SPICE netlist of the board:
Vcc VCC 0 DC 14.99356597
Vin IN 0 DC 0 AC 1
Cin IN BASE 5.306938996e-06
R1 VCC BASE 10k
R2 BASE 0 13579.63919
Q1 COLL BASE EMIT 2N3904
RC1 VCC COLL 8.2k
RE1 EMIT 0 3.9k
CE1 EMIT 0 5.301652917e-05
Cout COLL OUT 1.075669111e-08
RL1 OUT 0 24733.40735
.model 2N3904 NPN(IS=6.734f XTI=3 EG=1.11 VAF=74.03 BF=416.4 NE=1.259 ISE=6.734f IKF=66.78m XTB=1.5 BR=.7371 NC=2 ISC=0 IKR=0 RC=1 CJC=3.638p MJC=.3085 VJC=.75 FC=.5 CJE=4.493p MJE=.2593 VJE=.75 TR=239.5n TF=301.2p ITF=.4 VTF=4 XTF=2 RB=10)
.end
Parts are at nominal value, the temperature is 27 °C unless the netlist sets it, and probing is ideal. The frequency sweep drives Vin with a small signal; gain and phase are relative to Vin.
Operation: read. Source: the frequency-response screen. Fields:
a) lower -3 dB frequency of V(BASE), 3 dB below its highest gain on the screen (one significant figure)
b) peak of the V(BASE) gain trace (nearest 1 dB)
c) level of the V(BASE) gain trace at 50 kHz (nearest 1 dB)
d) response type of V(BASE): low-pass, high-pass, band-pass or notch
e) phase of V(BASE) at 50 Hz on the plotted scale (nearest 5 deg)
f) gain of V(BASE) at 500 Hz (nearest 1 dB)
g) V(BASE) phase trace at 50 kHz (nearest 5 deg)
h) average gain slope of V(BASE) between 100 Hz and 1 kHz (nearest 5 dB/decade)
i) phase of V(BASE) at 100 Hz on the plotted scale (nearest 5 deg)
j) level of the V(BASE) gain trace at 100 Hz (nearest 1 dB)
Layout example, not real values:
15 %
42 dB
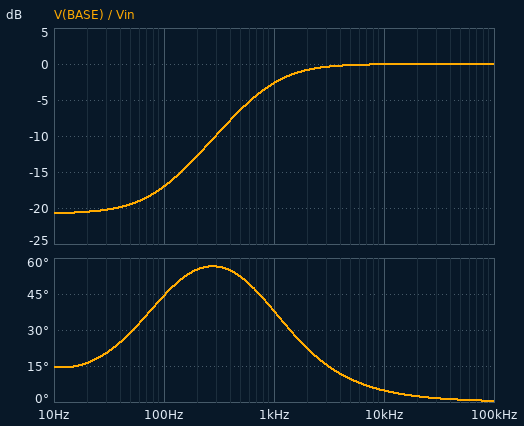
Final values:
900 Hz
0 dB
0 dB
high-pass
30 deg
-6 dB
0 deg
15 dB/decade
45 deg
-17 dB
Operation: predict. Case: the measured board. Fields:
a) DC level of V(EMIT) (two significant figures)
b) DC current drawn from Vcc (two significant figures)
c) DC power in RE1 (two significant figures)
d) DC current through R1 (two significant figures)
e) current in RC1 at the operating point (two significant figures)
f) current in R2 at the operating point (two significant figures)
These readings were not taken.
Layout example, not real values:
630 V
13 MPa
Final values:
5.8 V
2.0 mA
8.6 mW
850 µA
1.1 mA
480 µA
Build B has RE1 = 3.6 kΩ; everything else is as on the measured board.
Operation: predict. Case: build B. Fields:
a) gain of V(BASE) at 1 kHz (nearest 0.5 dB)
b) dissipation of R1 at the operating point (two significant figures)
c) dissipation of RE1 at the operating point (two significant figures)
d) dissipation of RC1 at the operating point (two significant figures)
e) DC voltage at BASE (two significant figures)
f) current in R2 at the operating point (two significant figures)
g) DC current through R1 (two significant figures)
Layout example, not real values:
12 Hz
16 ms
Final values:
-3.0 dB
7.6 mW
8.7 mW
11 mW
6.3 V
460 µA
870 µA
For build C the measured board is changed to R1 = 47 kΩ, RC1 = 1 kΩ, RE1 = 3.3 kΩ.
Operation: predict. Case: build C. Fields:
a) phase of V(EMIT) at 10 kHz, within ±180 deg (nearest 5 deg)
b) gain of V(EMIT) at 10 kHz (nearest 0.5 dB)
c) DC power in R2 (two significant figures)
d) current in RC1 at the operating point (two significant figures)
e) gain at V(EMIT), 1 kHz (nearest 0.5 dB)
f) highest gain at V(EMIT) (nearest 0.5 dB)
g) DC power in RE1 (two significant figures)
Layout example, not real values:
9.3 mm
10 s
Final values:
-90 deg
-41.0 dB
800 µW
800 µA
-21.0 dB
-1.0 dB
2.1 mW
